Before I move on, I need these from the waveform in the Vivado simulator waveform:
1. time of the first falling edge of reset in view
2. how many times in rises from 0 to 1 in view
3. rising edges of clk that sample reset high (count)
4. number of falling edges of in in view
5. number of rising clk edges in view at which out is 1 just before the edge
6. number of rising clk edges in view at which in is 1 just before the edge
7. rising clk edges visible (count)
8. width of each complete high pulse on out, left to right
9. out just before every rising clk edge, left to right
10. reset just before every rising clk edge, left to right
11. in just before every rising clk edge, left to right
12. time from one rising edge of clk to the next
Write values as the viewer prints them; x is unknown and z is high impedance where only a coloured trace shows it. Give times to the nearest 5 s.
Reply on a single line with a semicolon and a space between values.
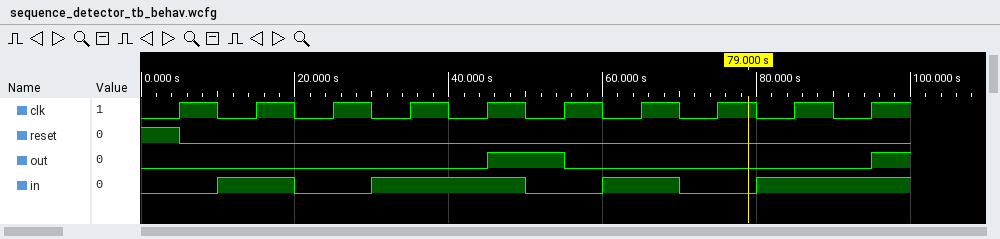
5 s; 4; 1; 3; 1; 6; 10; 10 s; 0 0 0 0 0 1 0 0 0 0; 1 0 0 0 0 0 0 0 0 0; 0 1 0 1 1 0 1 0 1 1; 10 s
